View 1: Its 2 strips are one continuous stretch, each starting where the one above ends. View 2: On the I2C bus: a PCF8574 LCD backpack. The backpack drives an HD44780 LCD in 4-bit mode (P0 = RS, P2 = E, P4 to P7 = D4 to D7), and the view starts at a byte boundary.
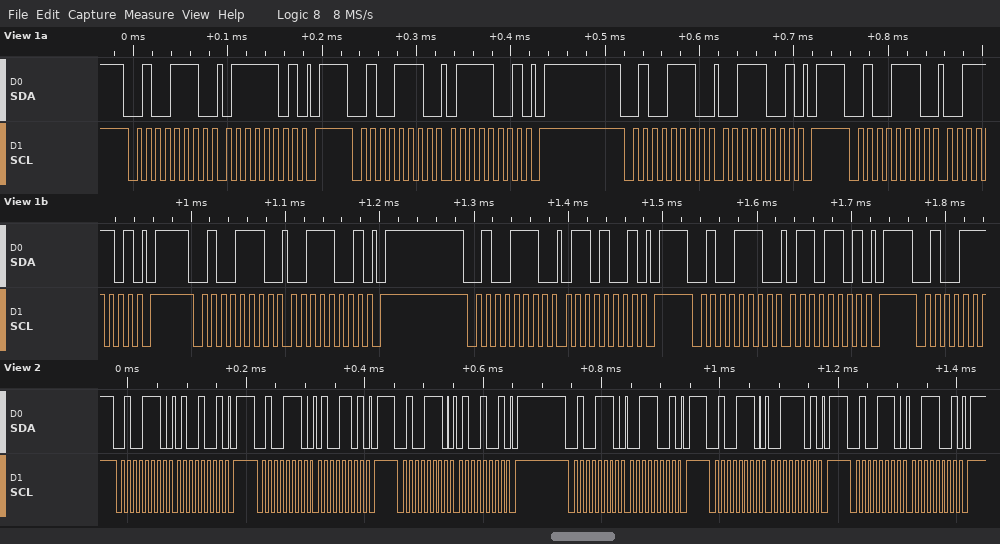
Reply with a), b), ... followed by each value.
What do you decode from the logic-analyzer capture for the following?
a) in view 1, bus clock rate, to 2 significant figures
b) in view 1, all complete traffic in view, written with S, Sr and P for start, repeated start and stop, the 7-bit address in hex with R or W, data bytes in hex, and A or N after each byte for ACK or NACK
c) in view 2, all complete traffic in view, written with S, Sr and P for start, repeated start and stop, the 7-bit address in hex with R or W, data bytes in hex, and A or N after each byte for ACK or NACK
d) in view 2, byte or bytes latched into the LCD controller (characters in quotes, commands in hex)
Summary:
a) 100 kHz
b) S 27W A 7D A P S 27W A 79 A P S 27W A 39 A P S 27W A 3D A P S 27W A 39 A P S 27W A 69 A P S 27W A 6D A P
c) S 27W A 49 A P S 27W A 4D A P S 27W A 49 A P S 27W A 39 A P S 27W A 3D A P S 27W A 39 A P
d) 'C'
